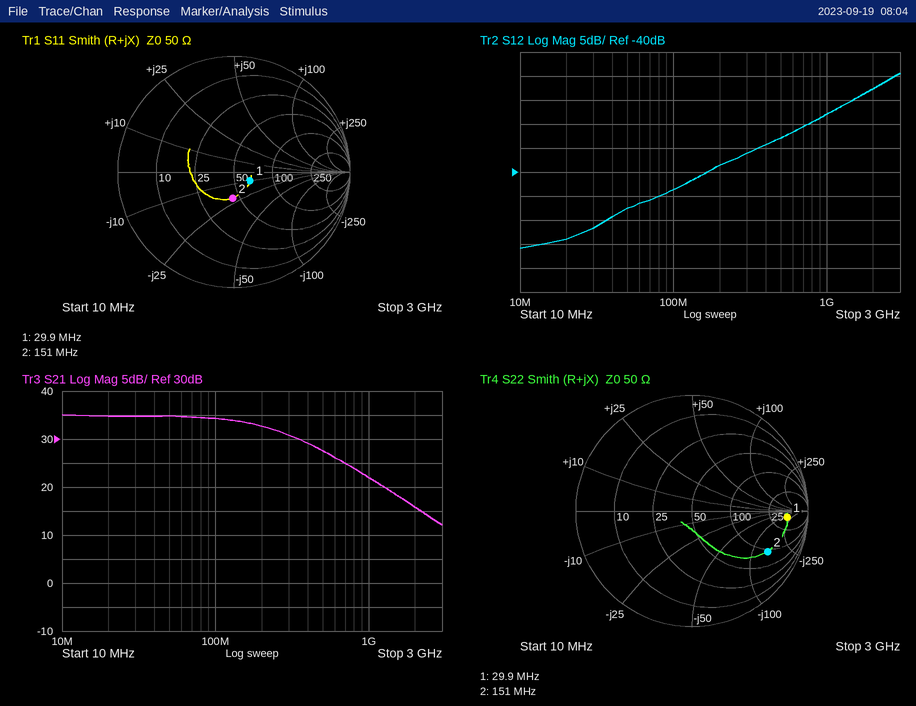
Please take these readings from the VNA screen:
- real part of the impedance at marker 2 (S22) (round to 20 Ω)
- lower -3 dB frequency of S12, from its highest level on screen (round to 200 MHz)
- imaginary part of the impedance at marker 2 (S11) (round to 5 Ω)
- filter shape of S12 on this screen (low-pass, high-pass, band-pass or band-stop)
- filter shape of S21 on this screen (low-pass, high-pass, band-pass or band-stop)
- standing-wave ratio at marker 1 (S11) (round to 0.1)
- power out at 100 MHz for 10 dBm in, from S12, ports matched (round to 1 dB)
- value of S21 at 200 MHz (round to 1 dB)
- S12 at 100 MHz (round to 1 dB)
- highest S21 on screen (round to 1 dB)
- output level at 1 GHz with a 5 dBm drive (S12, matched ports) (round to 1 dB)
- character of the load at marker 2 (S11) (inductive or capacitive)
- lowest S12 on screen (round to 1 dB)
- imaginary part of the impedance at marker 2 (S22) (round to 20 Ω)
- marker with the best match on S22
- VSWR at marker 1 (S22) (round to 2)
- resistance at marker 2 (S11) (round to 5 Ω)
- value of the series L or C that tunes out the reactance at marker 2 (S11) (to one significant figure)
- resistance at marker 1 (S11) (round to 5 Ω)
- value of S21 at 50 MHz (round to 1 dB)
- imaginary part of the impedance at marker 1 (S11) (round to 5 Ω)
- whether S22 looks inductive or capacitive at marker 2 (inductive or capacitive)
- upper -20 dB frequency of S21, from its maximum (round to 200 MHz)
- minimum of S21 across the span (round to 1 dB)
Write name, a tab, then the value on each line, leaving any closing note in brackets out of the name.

real part of the impedance at marker 2 (S22)	100 Ω
lower -3 dB frequency of S12, from its highest level on screen	2.0 GHz
imaginary part of the impedance at marker 2 (S11)	-20 Ω
filter shape of S12 on this screen	high-pass
filter shape of S21 on this screen	low-pass
standing-wave ratio at marker 1 (S11)	1.4
power out at 100 MHz for 10 dBm in, from S12, ports matched	-34 dBm
value of S21 at 200 MHz	33 dB
S12 at 100 MHz	-44 dB
highest S21 on screen	35 dB
output level at 1 GHz with a 5 dBm drive (S12, matched ports)	-23 dBm
character of the load at marker 2 (S11)	capacitive
lowest S12 on screen	-56 dB
imaginary part of the impedance at marker 2 (S22)	-140 Ω
marker with the best match on S22	marker 2
VSWR at marker 1 (S22)	10
resistance at marker 2 (S11)	45 Ω
value of the series L or C that tunes out the reactance at marker 2 (S11)	20 nH
resistance at marker 1 (S11)	65 Ω
value of S21 at 50 MHz	35 dB
imaginary part of the impedance at marker 1 (S11)	-10 Ω
whether S22 looks inductive or capacitive at marker 2	capacitive
upper -20 dB frequency of S21, from its maximum	2.2 GHz
minimum of S21 across the span	12 dB
